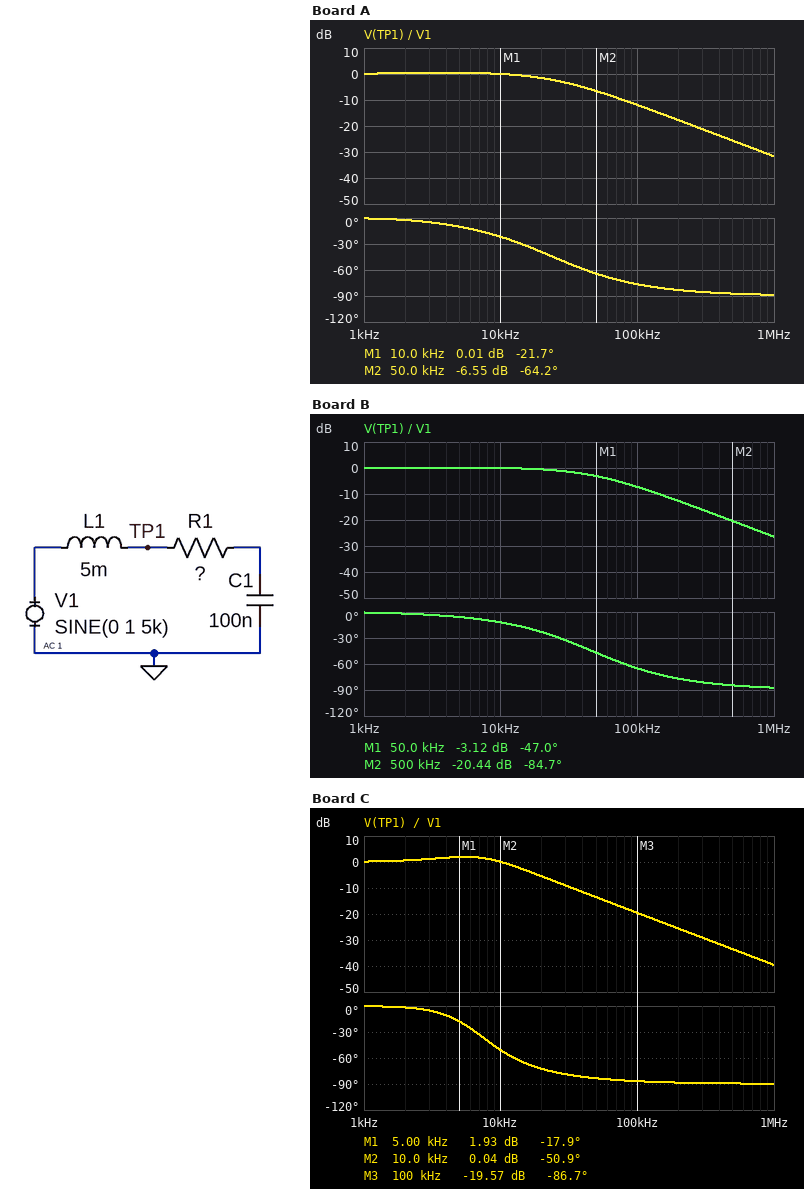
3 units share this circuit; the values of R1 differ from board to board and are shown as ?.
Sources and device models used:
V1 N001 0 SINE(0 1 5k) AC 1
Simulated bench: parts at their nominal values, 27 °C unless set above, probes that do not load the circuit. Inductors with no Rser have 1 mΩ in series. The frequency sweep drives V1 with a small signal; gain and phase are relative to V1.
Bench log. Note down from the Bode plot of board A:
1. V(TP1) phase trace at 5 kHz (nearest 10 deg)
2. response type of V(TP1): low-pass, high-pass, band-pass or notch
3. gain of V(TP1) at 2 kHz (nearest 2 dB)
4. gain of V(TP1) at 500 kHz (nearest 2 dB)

-10 deg
low-pass
0 dB
-26 dB
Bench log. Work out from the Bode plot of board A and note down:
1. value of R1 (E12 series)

820 Ω
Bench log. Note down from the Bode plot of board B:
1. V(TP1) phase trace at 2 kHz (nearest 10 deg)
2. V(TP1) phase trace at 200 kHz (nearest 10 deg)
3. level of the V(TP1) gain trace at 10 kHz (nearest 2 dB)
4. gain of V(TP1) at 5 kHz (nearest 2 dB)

0 deg
-80 deg
0 dB
0 dB
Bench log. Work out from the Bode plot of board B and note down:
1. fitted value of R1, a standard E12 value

1.5 kΩ
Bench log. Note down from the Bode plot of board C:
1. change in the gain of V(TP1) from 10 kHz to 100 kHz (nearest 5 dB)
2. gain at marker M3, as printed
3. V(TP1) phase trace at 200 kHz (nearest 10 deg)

-20 dB
-19.57 dB
-90 deg
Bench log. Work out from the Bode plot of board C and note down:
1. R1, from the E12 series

330 Ω
